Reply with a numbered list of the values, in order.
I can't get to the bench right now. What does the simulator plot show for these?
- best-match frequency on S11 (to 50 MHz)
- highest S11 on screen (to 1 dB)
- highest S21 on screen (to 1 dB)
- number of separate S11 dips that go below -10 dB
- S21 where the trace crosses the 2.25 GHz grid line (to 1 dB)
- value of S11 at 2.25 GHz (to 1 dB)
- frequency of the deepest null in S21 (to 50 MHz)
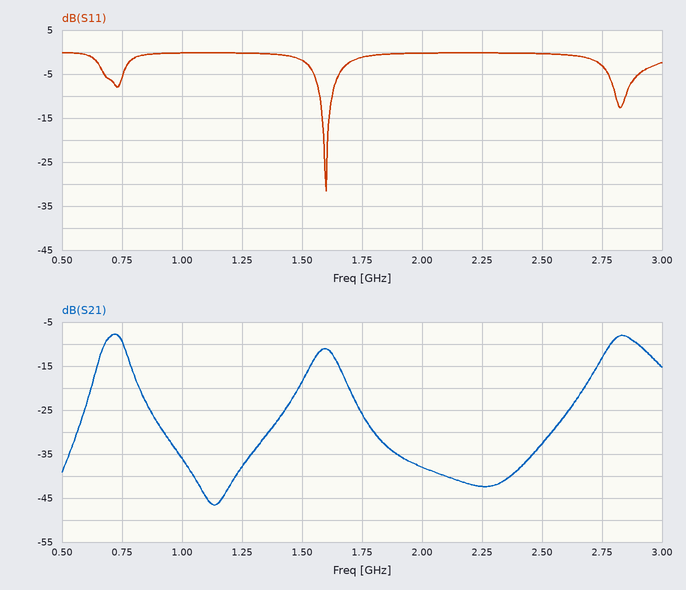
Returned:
1. 1.60 GHz
2. 0 dB
3. -8 dB
4. 2
5. -42 dB
6. 0 dB
7. 1.15 GHz
